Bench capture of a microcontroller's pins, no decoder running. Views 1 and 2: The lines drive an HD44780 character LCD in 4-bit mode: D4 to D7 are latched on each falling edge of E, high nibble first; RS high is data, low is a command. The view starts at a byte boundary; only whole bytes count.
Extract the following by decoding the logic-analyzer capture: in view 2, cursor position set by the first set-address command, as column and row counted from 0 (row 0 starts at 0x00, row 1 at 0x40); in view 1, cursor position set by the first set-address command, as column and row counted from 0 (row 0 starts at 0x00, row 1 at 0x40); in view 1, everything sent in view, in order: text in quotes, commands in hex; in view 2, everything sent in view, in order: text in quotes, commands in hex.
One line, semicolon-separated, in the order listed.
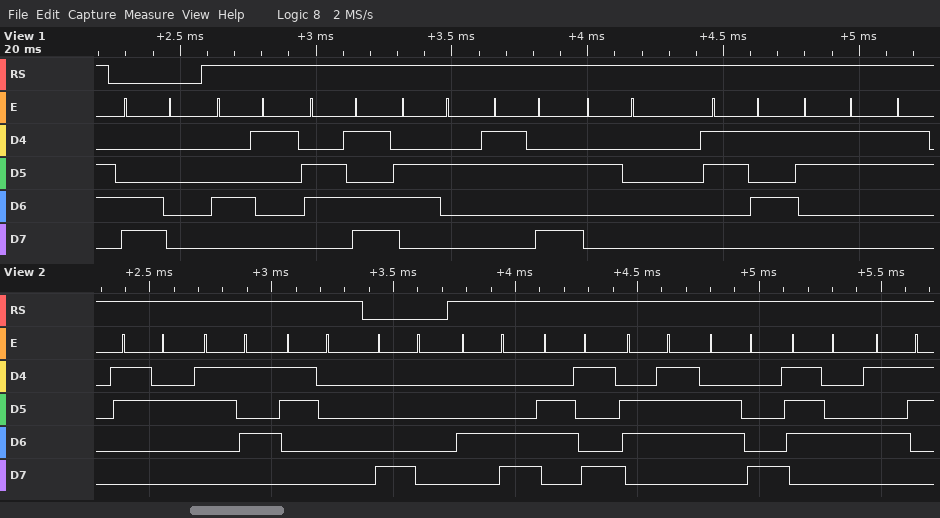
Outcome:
column 0, row 0; column 0, row 1; 0xC0 "Amb: 53"; "250" 0x80 "LightS"
